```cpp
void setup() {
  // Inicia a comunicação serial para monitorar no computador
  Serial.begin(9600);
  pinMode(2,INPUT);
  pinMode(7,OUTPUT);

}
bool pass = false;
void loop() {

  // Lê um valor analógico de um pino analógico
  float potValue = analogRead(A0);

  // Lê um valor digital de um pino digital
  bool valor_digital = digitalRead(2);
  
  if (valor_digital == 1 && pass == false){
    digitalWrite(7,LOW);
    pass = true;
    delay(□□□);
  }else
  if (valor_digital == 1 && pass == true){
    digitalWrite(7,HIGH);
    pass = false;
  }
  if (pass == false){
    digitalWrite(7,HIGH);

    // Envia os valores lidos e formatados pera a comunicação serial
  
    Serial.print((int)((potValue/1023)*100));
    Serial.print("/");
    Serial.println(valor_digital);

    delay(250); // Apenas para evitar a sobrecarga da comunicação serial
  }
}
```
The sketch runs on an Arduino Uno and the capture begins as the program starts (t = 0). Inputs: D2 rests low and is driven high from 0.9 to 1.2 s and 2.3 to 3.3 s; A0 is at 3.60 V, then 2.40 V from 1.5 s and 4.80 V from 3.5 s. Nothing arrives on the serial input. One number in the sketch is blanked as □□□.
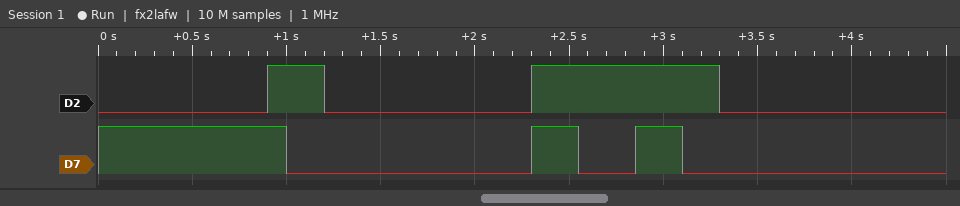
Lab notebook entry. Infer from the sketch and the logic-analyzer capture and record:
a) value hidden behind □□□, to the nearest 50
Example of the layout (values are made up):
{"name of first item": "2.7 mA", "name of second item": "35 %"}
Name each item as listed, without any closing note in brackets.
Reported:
{"value hidden behind □□□, to the nearest 50": "300"}
